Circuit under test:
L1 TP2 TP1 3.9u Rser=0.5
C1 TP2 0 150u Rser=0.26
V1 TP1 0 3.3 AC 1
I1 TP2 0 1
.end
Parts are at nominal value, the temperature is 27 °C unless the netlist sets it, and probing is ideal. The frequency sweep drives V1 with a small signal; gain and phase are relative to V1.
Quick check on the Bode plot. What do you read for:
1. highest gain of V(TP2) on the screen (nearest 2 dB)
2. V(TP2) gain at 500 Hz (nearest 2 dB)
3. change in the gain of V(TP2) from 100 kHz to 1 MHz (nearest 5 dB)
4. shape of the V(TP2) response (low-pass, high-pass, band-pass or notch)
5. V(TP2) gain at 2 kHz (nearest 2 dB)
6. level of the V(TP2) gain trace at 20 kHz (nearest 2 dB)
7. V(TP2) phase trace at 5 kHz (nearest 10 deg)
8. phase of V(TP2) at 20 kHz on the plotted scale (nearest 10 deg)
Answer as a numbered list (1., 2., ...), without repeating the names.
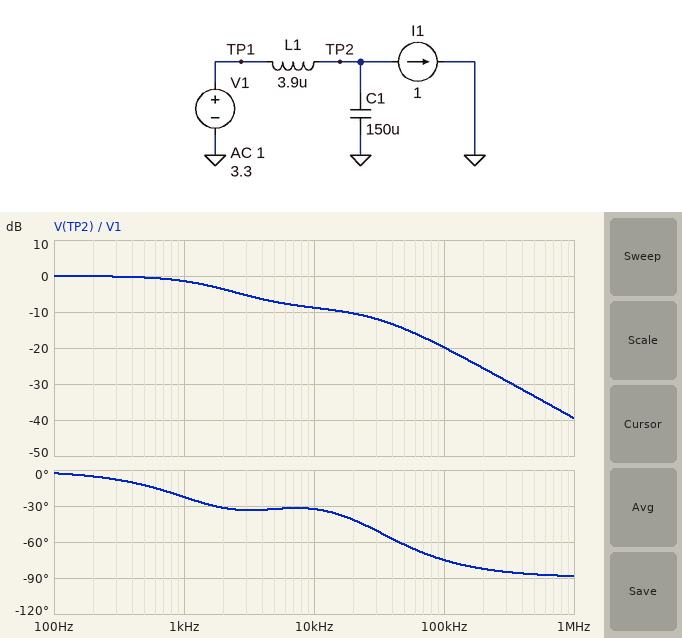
1. 0 dB
2. 0 dB
3. -20 dB
4. low-pass
5. -4 dB
6. -10 dB
7. -30 deg
8. -40 deg
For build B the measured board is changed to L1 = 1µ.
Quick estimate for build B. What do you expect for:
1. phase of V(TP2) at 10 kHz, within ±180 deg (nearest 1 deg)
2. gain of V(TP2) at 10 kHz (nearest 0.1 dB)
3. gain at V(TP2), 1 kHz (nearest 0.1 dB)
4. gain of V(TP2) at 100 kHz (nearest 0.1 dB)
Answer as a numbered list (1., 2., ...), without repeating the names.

1. -19 deg
2. -8.7 dB
3. -1.5 dB
4. -11.5 dB
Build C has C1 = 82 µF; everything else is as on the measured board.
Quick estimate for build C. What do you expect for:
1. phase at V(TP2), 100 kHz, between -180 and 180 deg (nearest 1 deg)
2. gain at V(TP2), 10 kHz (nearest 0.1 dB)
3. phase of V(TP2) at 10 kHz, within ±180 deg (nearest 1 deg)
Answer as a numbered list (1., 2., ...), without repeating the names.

1. -77 deg
2. -7.4 dB
3. -41 deg
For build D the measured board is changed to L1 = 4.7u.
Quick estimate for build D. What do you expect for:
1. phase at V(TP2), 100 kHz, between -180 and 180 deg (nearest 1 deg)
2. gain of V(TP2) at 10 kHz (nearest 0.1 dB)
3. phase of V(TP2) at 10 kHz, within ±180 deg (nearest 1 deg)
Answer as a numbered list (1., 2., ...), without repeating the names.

1. -78 deg
2. -8.9 dB
3. -36 deg
